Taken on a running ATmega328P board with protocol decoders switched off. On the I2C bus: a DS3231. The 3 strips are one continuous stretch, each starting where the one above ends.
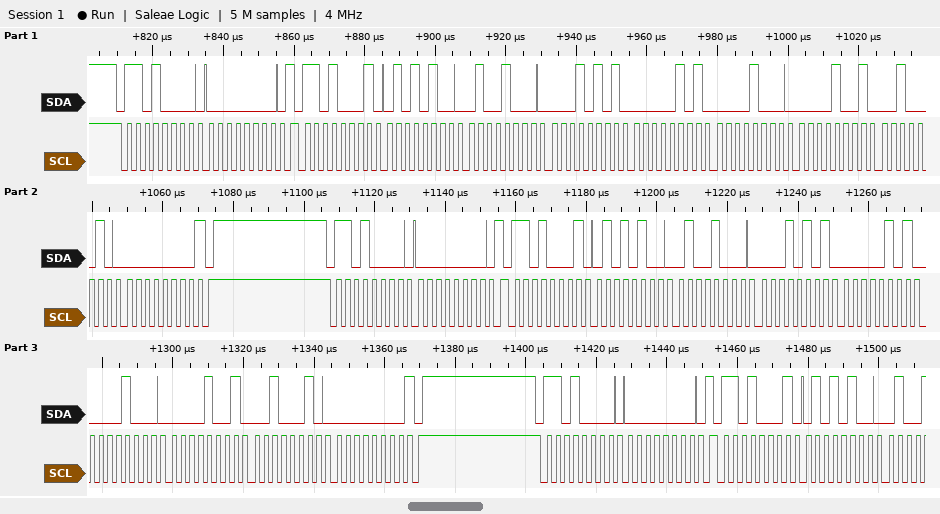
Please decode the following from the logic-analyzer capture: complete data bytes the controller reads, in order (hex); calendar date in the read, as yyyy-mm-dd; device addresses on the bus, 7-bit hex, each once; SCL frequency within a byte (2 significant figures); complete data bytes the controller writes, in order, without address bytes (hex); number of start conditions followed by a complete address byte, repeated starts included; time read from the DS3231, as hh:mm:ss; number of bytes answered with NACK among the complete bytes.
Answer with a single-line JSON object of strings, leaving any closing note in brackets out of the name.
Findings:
{"complete data bytes the controller reads, in order": "54 48 15 05 08 09 22 00 54 48 15 05 08 09 22 00 54", "calendar date in the read, as yyyy-mm-dd": "2022-09-08", "device addresses on the bus, 7-bit hex, each once": "0x68", "SCL frequency within a byte": "400 kHz", "complete data bytes the controller writes, in order, without address bytes": "00 00 00", "number of start conditions followed by a complete address byte, repeated starts included": "6", "time read from the DS3231, as hh:mm:ss": "15:48:54", "number of bytes answered with NACK among the complete bytes": "2"}
